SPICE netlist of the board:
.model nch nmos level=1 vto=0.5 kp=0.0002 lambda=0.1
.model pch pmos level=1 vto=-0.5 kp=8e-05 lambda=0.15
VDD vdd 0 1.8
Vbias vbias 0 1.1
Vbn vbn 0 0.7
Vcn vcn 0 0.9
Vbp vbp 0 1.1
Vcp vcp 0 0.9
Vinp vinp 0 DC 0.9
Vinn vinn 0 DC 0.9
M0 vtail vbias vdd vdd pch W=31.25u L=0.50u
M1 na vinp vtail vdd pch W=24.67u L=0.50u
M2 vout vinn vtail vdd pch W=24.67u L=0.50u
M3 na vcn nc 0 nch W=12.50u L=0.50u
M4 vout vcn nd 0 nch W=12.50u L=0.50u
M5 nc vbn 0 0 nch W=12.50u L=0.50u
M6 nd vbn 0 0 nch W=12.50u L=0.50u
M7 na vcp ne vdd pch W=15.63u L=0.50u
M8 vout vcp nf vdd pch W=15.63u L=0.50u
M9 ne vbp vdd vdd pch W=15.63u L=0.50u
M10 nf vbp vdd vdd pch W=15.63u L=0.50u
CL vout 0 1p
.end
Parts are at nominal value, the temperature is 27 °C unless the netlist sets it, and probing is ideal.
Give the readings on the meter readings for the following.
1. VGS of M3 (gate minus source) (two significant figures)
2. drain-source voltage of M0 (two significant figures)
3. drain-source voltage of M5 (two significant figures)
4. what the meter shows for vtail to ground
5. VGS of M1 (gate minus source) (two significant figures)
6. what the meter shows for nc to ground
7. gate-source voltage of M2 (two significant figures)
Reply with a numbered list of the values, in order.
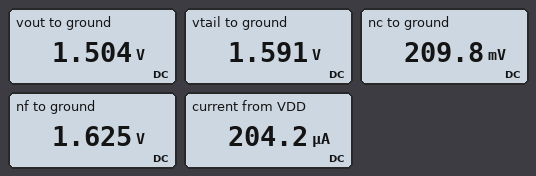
1. 690 mV
2. -210 mV
3. 210 mV
4. 1.591 V
5. -690 mV
6. 209.8 mV
7. -690 mV
